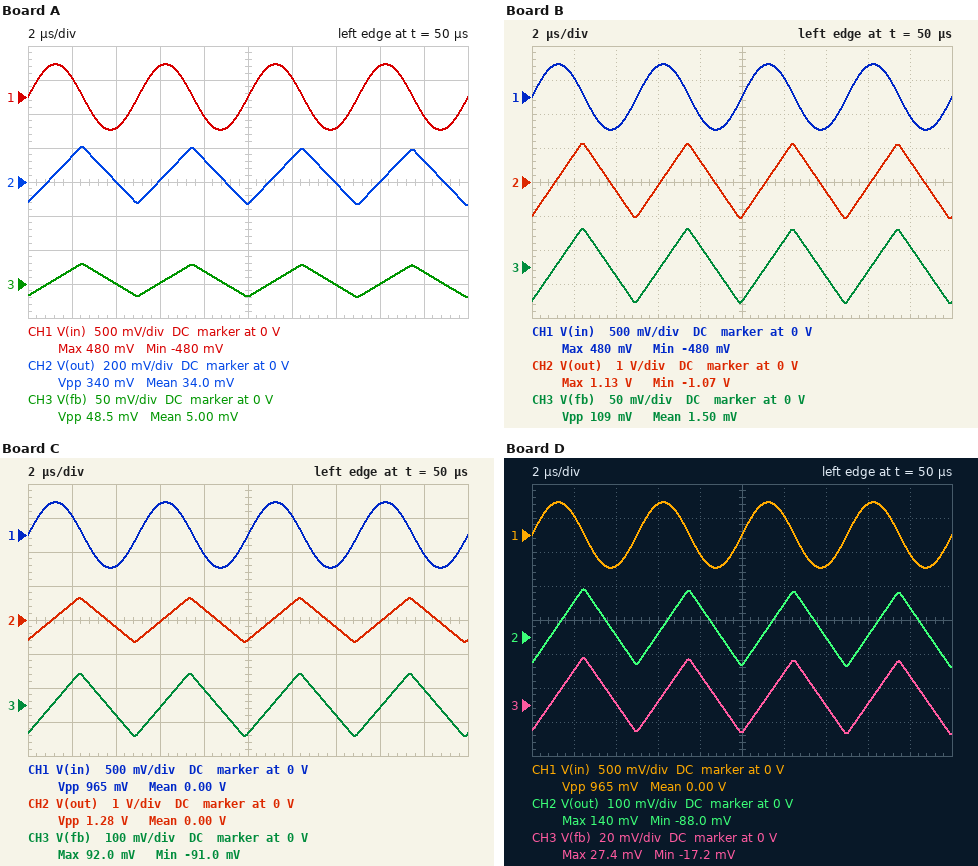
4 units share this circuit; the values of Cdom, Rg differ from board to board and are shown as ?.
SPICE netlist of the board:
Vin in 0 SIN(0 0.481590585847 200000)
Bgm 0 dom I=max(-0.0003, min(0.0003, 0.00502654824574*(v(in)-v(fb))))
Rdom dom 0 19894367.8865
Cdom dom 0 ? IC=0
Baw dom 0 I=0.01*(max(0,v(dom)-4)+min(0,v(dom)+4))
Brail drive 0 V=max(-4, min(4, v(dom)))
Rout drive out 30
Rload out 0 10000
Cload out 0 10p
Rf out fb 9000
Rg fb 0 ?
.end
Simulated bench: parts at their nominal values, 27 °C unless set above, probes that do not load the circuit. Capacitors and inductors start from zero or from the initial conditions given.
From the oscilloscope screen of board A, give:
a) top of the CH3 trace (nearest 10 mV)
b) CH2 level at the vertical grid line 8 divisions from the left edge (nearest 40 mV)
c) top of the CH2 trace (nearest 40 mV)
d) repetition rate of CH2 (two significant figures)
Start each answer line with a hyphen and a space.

- 30 mV
- 0 V
- 200 mV
- 200 kHz
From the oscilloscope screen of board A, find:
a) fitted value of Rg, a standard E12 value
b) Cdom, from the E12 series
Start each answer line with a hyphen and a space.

- 1.5 kΩ
- 2.2 nF
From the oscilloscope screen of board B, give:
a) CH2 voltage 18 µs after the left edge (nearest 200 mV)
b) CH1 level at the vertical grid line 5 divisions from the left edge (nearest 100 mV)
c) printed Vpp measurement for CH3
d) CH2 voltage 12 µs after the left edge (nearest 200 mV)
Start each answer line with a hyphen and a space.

- 600 mV
- 0 V
- 109 mV
- 800 mV
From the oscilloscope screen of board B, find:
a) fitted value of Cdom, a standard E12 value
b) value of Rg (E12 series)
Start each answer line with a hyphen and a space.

- 330 pF
- 470 Ω
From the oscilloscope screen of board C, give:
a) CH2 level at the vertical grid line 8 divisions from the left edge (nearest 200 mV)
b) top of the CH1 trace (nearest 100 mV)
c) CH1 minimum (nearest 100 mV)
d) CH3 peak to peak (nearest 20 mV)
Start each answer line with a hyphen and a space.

- 0 V
- 500 mV
- -500 mV
- 180 mV
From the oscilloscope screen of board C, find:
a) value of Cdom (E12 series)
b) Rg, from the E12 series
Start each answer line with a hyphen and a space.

- 560 pF
- 1.5 kΩ
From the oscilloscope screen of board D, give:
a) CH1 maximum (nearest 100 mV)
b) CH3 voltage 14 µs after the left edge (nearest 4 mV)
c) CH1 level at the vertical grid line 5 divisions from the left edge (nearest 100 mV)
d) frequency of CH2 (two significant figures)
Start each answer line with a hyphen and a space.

- 500 mV
- 0 V
- 0 V
- 200 kHz
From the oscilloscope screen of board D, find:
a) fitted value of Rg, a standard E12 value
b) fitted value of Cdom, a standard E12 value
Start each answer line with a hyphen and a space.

- 2.2 kΩ
- 3.3 nF
